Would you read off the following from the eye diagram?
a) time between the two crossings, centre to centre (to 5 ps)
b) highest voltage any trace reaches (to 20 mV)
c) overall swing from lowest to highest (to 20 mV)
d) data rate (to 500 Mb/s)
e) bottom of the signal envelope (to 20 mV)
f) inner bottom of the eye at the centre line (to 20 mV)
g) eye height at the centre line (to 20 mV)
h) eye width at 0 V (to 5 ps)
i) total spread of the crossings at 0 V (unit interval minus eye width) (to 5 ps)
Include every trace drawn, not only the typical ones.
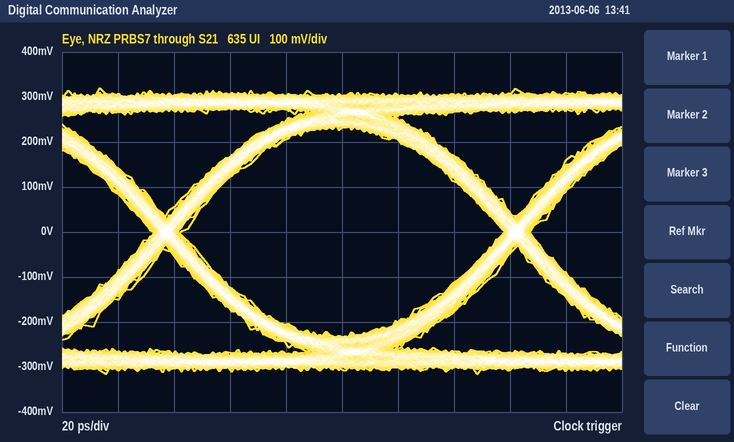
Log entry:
125 ps
320 mV
640 mV
8.0 Gb/s
-320 mV
-240 mV
460 mV
115 ps
10 ps
